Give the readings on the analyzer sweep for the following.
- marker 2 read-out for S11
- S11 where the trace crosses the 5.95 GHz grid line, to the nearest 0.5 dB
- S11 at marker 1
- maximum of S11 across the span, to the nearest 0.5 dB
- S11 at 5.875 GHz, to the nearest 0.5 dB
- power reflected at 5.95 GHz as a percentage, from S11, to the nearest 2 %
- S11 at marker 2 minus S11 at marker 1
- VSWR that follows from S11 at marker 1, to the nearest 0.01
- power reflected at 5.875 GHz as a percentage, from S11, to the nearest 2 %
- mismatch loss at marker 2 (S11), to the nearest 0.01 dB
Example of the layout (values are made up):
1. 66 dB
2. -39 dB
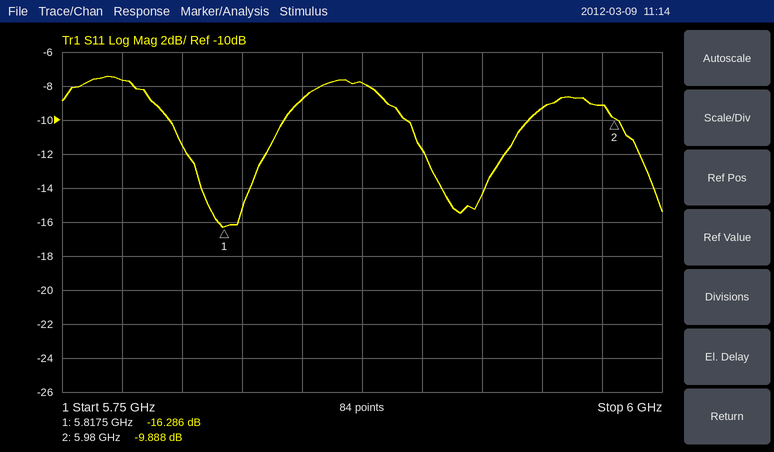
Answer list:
1. -9.888 dB
2. -9.5 dB
3. -16.286 dB
4. -7.5 dB
5. -8.0 dB
6. 12 %
7. 6.398 dB
8. 1.36
9. 16 %
10. 0.47 dB
